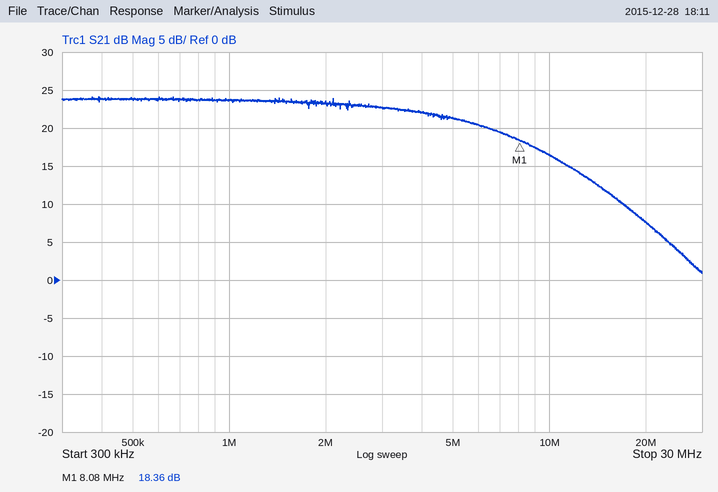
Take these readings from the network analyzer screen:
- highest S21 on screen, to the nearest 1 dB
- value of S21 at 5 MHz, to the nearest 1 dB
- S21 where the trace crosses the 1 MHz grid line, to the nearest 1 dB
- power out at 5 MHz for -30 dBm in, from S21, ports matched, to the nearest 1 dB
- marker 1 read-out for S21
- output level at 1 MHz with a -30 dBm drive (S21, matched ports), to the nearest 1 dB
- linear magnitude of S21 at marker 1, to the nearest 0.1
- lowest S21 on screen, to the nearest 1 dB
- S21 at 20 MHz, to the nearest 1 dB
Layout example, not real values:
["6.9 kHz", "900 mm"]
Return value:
["24 dB", "21 dB", "24 dB", "-9 dBm", "18.36 dB", "-6 dBm", "8.3", "1 dB", "8 dB"]
